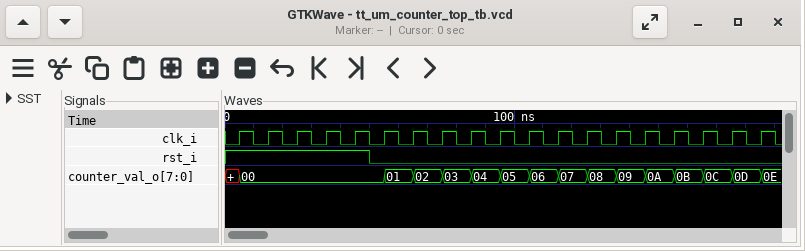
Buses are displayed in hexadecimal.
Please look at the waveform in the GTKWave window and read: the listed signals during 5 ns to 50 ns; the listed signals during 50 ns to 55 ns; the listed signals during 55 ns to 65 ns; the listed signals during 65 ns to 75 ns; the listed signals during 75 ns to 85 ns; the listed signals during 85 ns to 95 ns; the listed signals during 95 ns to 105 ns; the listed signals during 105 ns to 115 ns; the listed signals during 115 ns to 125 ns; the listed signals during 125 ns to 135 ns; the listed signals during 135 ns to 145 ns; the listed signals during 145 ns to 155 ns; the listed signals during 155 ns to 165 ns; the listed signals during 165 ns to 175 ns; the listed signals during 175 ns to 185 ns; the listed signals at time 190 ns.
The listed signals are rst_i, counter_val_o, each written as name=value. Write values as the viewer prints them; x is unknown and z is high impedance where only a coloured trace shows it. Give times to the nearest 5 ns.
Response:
rst_i=1, counter_val_o=00
rst_i=0, counter_val_o=00
rst_i=0, counter_val_o=01
rst_i=0, counter_val_o=02
rst_i=0, counter_val_o=03
rst_i=0, counter_val_o=04
rst_i=0, counter_val_o=05
rst_i=0, counter_val_o=06
rst_i=0, counter_val_o=07
rst_i=0, counter_val_o=08
rst_i=0, counter_val_o=09
rst_i=0, counter_val_o=0A
rst_i=0, counter_val_o=0B
rst_i=0, counter_val_o=0C
rst_i=0, counter_val_o=0D
rst_i=0, counter_val_o=0E
